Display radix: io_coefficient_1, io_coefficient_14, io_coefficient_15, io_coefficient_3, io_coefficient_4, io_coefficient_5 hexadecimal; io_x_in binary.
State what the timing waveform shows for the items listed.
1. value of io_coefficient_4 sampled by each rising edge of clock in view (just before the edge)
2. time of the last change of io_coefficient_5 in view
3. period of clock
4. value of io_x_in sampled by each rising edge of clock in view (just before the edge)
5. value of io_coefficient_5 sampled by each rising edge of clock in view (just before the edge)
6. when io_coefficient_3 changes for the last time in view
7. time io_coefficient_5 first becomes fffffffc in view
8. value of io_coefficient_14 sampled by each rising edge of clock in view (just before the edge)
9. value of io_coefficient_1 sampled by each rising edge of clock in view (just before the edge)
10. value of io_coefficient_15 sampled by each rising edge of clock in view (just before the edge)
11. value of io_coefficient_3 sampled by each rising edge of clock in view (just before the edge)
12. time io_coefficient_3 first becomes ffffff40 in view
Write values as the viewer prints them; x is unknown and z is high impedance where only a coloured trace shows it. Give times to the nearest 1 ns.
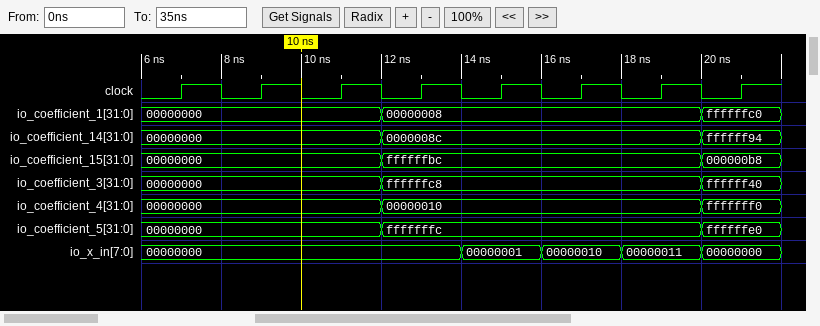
00000000, 00000000, 00000000, 00000010, 00000010, 00000010, 00000010, fffffff0
20 ns
2 ns
00000000, 00000000, 00000000, 00000000, 00000001, 00000010, 00000011, 00000000
00000000, 00000000, 00000000, fffffffc, fffffffc, fffffffc, fffffffc, ffffffe0
20 ns
12 ns
00000000, 00000000, 00000000, 0000008c, 0000008c, 0000008c, 0000008c, ffffff94
00000000, 00000000, 00000000, 00000008, 00000008, 00000008, 00000008, ffffffc0
00000000, 00000000, 00000000, ffffffbc, ffffffbc, ffffffbc, ffffffbc, 000000b8
00000000, 00000000, 00000000, ffffffc8, ffffffc8, ffffffc8, ffffffc8, ffffff40
20 ns
